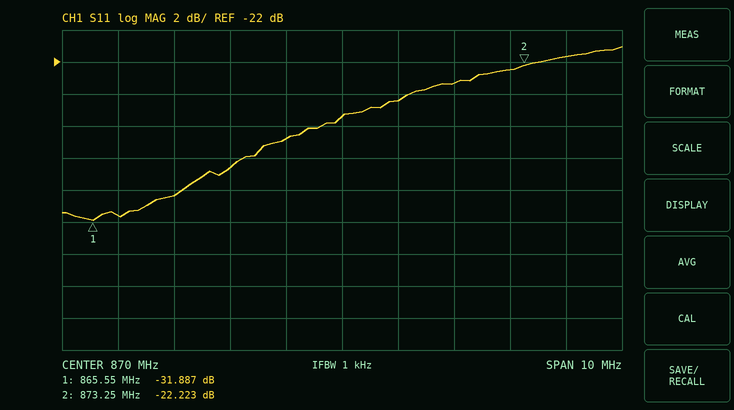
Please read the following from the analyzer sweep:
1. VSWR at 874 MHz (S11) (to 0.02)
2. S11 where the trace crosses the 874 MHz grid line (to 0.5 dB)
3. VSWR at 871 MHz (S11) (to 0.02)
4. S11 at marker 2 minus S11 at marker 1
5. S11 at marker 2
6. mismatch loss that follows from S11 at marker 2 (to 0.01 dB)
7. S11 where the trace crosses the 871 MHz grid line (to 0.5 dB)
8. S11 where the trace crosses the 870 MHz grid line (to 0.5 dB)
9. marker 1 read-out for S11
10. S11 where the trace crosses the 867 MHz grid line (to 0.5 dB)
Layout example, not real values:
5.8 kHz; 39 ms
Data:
1.18; -21.5 dB; 1.12; 9.664 dB; -22.223 dB; 0.03 dB; -24.5 dB; -25.5 dB; -31.887 dB; -30.5 dB
